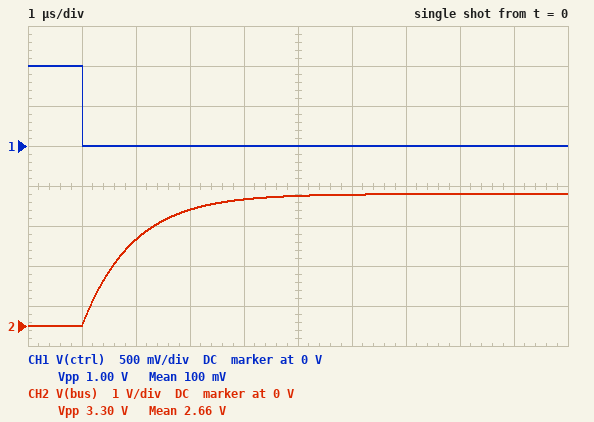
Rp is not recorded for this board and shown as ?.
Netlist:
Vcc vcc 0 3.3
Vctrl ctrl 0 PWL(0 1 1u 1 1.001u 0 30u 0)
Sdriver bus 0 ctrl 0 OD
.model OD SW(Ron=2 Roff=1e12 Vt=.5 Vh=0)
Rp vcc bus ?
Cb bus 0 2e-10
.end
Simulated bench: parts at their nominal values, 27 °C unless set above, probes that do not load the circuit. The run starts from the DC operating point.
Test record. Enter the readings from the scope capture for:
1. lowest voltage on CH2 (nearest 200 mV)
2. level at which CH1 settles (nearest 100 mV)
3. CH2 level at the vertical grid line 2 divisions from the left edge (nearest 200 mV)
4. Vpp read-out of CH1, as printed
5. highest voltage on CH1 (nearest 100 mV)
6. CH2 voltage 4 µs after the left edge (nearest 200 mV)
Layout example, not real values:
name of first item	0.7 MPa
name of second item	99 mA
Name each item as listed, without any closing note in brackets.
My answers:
lowest voltage on CH2	0 V
level at which CH1 settles	0 V
CH2 level at the vertical grid line 2 divisions from the left edge	2.2 V
Vpp read-out of CH1, as printed	1.00 V
highest voltage on CH1	1.0 V
CH2 voltage 4 µs after the left edge	3.2 V
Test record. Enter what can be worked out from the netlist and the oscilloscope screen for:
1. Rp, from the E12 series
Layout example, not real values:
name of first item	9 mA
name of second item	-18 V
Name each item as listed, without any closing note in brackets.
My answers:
Rp, from the E12 series	4.7 kΩ
